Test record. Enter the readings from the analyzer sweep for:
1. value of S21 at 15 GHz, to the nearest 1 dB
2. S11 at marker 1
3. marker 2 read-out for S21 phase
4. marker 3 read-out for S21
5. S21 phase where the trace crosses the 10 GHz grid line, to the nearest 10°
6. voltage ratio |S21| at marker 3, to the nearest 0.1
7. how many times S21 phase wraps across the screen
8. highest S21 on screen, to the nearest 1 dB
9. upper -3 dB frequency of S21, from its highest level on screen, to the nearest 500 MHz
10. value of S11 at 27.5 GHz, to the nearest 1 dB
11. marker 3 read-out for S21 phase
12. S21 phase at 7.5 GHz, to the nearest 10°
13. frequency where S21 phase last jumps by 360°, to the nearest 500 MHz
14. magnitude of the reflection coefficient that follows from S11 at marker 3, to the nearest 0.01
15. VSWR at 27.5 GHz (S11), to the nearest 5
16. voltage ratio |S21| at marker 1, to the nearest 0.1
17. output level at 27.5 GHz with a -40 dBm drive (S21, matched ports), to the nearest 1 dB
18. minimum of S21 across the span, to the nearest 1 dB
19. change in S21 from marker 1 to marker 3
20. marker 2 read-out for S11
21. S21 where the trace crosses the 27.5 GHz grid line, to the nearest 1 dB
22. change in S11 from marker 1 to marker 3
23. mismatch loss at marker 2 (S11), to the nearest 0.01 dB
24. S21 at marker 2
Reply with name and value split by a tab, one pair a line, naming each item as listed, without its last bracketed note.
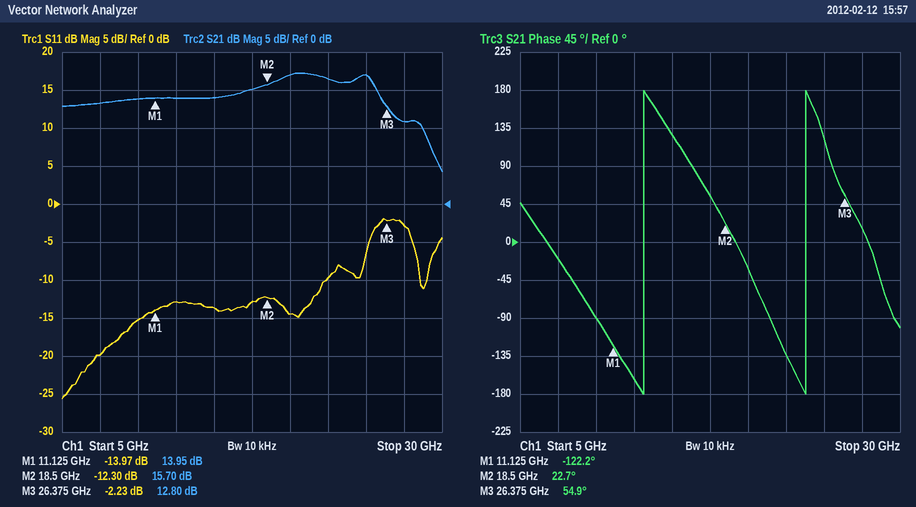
value of S21 at 15 GHz, to the nearest 1 dB	14 dB
S11 at marker 1	-13.97 dB
marker 2 read-out for S21 phase	22.7°
marker 3 read-out for S21	12.80 dB
S21 phase where the trace crosses the 10 GHz grid line, to the nearest 10°	-90°
voltage ratio |S21| at marker 3, to the nearest 0.1	4.4
how many times S21 phase wraps across the screen	2
highest S21 on screen, to the nearest 1 dB	17 dB
upper -3 dB frequency of S21, from its highest level on screen, to the nearest 500 MHz	26.0 GHz
value of S11 at 27.5 GHz, to the nearest 1 dB	-3 dB
marker 3 read-out for S21 phase	54.9°
S21 phase at 7.5 GHz, to the nearest 10°	-20°
frequency where S21 phase last jumps by 360°, to the nearest 500 MHz	24.0 GHz
magnitude of the reflection coefficient that follows from S11 at marker 3, to the nearest 0.01	0.77
VSWR at 27.5 GHz (S11), to the nearest 5	5
voltage ratio |S21| at marker 1, to the nearest 0.1	5.0
output level at 27.5 GHz with a -40 dBm drive (S21, matched ports), to the nearest 1 dB	-29 dBm
minimum of S21 across the span, to the nearest 1 dB	4 dB
change in S21 from marker 1 to marker 3	-1.15 dB
marker 2 read-out for S11	-12.30 dB
S21 where the trace crosses the 27.5 GHz grid line, to the nearest 1 dB	11 dB
change in S11 from marker 1 to marker 3	11.74 dB
mismatch loss at marker 2 (S11), to the nearest 0.01 dB	0.26 dB
S21 at marker 2	15.70 dB
